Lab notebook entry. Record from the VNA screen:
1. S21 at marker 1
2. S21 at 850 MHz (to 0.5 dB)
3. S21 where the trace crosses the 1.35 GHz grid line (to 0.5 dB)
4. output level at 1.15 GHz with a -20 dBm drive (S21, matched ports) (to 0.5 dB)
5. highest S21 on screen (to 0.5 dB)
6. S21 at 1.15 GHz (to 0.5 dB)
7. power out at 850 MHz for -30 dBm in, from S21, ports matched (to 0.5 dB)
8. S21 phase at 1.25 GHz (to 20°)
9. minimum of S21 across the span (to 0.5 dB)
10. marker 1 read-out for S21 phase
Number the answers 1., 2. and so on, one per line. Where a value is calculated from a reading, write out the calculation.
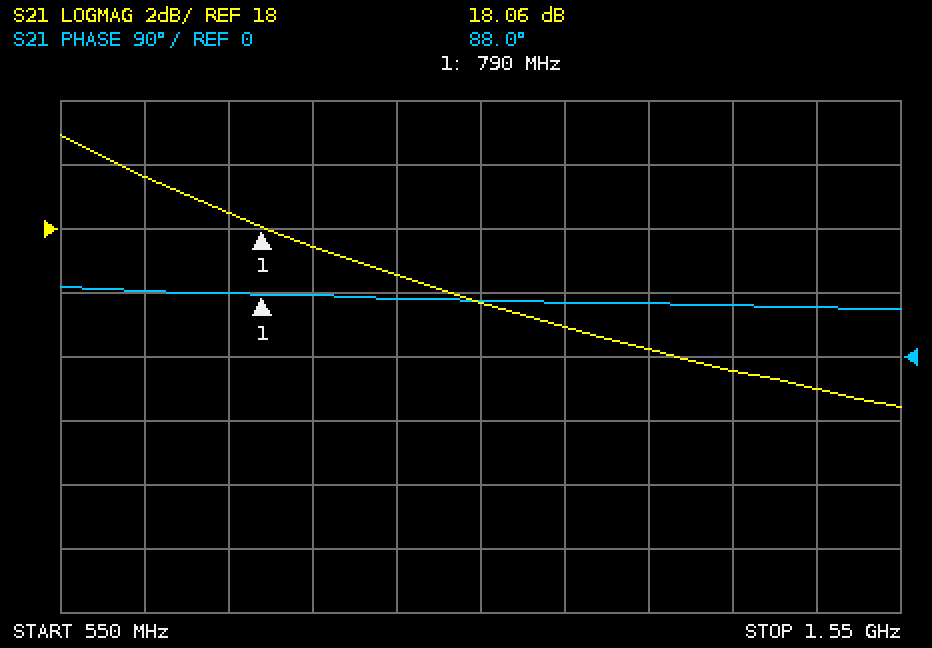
1. 18.06 dB
2. 17.5 dB
3. 13.5 dB
4. -20 dBm + (15.0 dB) = -5.0 dBm
5. 21.0 dB
6. 15.0 dB
7. -30 dBm + (17.5 dB) = -12.5 dBm
8. 80°
9. 12.5 dB
10. 88.0°
